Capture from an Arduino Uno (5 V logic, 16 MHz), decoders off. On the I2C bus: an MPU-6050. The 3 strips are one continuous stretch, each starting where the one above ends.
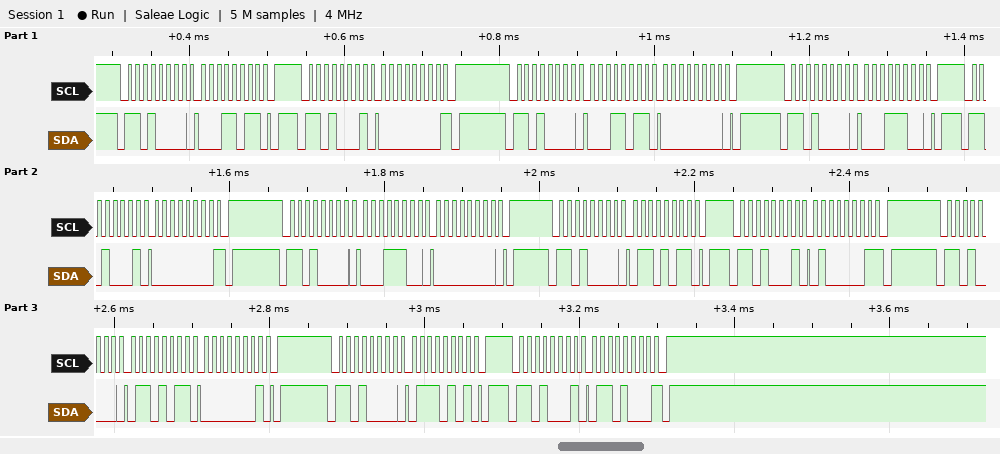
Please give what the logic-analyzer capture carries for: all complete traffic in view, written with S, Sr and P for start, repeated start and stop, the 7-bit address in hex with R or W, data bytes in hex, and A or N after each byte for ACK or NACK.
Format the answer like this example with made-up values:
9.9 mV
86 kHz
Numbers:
S 68W A 1B A P S 68R A 00 N P S 68W A 1B A 00 A P S 68W A 1C A P S 68R A 00 N P S 68W A 1C A 00 A P S 68W A 6B A P S 68R A 41 N P S 68W A 6B A 01 A P S 68W A 75 A P S 68R A 68 N P
